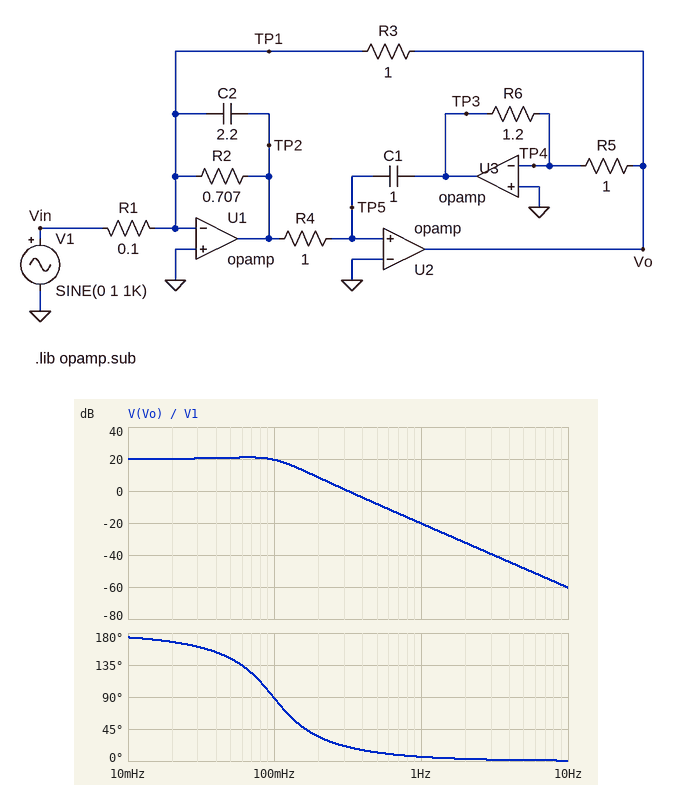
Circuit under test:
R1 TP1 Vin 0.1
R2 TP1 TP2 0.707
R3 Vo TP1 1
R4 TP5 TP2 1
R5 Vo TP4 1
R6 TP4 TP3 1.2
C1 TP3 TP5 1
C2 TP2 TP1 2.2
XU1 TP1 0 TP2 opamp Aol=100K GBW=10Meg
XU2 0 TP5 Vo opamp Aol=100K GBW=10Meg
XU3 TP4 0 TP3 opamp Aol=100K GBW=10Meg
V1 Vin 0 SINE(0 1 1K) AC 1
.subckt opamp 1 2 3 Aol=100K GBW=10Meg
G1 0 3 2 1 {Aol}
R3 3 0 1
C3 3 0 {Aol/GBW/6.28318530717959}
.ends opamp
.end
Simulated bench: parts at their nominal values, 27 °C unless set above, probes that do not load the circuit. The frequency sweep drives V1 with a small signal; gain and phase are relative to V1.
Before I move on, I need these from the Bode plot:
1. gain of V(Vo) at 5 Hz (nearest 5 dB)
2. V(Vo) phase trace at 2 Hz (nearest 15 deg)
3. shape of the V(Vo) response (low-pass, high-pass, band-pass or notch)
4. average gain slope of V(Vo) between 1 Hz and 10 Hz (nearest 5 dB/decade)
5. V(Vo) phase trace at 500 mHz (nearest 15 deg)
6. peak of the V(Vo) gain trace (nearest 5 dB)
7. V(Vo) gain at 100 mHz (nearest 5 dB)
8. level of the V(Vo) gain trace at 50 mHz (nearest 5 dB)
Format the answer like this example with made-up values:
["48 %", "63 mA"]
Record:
["-50 dB", "0 deg", "low-pass", "-40 dB/decade", "15 deg", "20 dB", "20 dB", "20 dB"]
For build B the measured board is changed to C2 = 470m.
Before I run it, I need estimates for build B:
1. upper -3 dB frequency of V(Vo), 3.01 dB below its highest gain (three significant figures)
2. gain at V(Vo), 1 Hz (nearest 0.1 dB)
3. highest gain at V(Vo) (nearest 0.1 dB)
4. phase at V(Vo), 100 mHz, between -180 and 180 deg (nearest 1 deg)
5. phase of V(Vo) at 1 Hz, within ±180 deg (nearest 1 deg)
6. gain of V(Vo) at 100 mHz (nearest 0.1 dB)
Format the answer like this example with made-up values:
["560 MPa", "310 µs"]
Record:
["115 mHz", "-7.5 dB", "20.0 dB", "126 deg", "27 deg", "17.6 dB"]
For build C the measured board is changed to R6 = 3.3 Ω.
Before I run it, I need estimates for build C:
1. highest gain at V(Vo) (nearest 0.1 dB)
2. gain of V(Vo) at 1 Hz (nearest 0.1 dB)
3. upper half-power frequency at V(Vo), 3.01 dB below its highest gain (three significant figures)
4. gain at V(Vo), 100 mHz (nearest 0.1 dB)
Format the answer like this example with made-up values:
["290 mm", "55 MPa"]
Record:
["20.0 dB", "-29.2 dB", "46.4 mHz", "9.2 dB"]
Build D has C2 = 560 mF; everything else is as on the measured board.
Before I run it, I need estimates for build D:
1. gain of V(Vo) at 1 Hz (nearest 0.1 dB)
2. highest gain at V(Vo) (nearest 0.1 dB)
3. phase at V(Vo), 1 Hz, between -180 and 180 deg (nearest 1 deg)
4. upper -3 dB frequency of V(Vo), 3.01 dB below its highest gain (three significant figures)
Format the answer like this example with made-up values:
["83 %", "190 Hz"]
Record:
["-8.8 dB", "20.0 dB", "23 deg", "119 mHz"]
